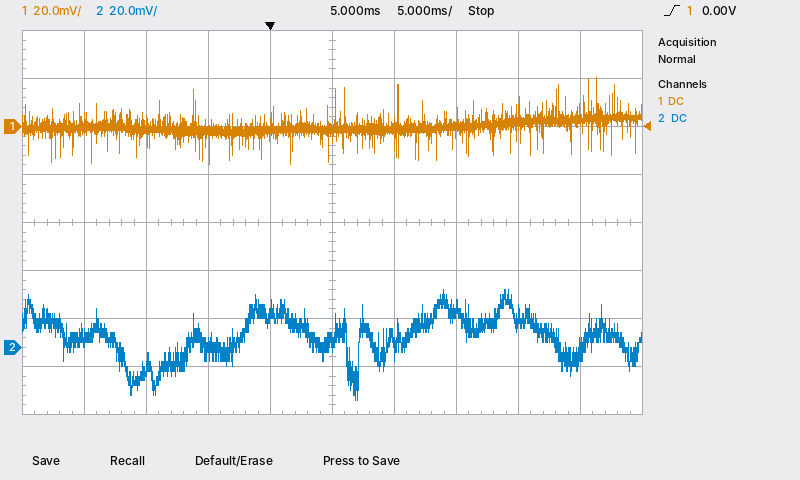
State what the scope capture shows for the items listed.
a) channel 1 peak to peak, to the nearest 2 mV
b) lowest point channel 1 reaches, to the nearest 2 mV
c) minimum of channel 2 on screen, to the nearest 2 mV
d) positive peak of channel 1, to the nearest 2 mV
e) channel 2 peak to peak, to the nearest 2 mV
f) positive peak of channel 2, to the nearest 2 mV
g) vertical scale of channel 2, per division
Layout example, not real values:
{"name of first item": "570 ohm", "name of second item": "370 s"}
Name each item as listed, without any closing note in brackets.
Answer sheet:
{"channel 1 peak to peak, to the nearest 2 mV": "36 mV", "lowest point channel 1 reaches, to the nearest 2 mV": "-16 mV", "minimum of channel 2 on screen, to the nearest 2 mV": "-22 mV", "positive peak of channel 1, to the nearest 2 mV": "20 mV", "channel 2 peak to peak, to the nearest 2 mV": "46 mV", "positive peak of channel 2, to the nearest 2 mV": "24 mV", "vertical scale of channel 2, per division": "20 mV"}
